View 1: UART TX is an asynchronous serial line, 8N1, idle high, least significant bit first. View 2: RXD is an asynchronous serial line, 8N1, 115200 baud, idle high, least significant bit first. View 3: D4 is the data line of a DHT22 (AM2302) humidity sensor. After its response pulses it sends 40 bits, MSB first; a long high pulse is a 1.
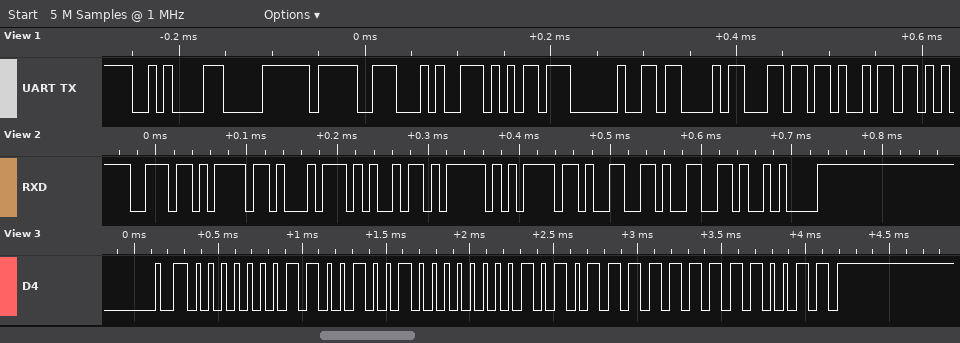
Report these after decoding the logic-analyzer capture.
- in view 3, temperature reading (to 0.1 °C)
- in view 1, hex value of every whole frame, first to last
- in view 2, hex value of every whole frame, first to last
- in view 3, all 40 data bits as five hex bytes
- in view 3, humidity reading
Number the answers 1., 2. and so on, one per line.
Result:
1. 35.1 °C
2. 0A F0 9F 94 B5 20 43 6C 69
3. 0x6E 0x6F 0x74 0x69 0x5F 0x6F 0x66 0x66 0x0A
4. 01 92 01 5F F3
5. 40.2 %
